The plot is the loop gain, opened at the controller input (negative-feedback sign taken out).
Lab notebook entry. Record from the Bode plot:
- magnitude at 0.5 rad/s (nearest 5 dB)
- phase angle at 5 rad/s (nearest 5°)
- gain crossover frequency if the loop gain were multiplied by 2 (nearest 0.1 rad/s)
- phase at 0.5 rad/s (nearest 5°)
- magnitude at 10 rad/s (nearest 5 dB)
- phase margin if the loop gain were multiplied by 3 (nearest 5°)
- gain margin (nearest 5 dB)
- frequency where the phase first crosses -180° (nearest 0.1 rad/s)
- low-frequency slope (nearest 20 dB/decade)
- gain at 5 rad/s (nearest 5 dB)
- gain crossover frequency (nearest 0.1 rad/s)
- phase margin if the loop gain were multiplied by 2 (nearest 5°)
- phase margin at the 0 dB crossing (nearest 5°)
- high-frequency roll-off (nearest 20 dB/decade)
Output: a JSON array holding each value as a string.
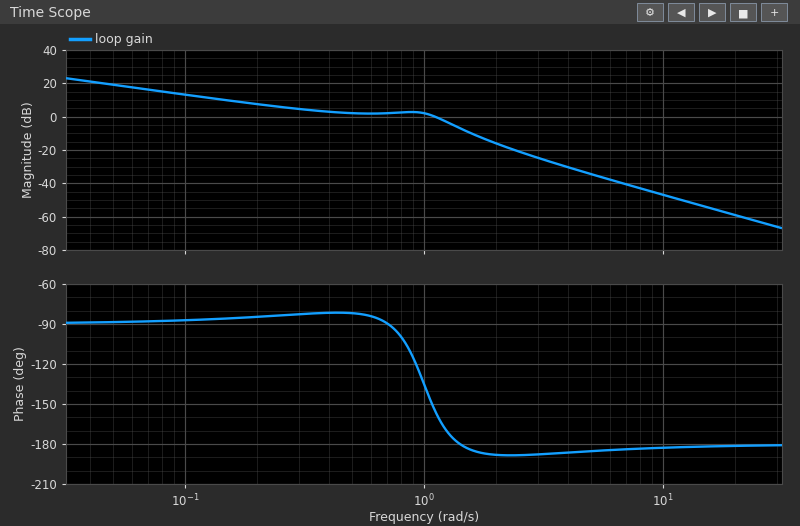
["0 dB", "-185°", "1.4 rad/s", "-80°", "-45 dB", "-5°", "5 dB", "1.4 rad/s", "-20 dB/decade", "-35 dB", "1.1 rad/s", "0°", "25°", "-40 dB/decade"]
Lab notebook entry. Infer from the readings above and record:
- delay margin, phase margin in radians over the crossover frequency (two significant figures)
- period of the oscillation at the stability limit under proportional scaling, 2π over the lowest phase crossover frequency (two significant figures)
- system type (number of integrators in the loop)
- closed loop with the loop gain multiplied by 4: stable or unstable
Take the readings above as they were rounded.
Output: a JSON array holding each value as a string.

["0.40 s", "4.5 s", "1", "unstable"]
